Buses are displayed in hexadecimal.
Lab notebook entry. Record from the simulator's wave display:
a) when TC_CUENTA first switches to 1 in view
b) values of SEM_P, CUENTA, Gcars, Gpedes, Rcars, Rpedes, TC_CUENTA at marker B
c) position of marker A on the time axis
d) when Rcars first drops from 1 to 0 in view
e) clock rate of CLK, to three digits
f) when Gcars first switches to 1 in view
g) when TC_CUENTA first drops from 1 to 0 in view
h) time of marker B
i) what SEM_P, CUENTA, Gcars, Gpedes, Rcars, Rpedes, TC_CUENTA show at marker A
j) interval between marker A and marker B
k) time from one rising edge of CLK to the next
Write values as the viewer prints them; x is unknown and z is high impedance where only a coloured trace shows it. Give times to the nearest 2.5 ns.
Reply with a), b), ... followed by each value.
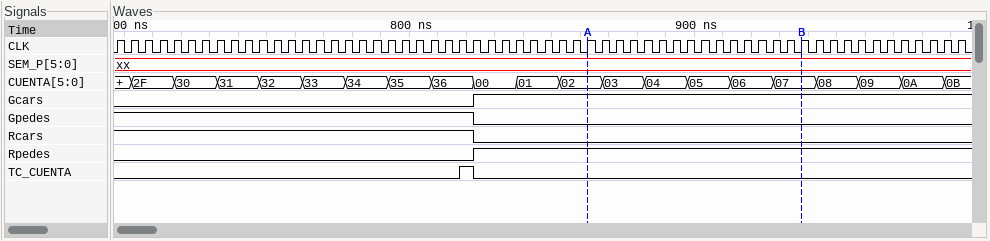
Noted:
a) 817.5 ns
b) SEM_P=xx, CUENTA=07, Gcars=1, Gpedes=0, Rcars=0, Rpedes=1, TC_CUENTA=0
c) 862.5 ns
d) 822.5 ns
e) 200 MHz
f) 822.5 ns
g) 822.5 ns
h) 937.5 ns
i) SEM_P=xx, CUENTA=02, Gcars=1, Gpedes=0, Rcars=0, Rpedes=1, TC_CUENTA=0
j) 75 ns
k) 5 ns
